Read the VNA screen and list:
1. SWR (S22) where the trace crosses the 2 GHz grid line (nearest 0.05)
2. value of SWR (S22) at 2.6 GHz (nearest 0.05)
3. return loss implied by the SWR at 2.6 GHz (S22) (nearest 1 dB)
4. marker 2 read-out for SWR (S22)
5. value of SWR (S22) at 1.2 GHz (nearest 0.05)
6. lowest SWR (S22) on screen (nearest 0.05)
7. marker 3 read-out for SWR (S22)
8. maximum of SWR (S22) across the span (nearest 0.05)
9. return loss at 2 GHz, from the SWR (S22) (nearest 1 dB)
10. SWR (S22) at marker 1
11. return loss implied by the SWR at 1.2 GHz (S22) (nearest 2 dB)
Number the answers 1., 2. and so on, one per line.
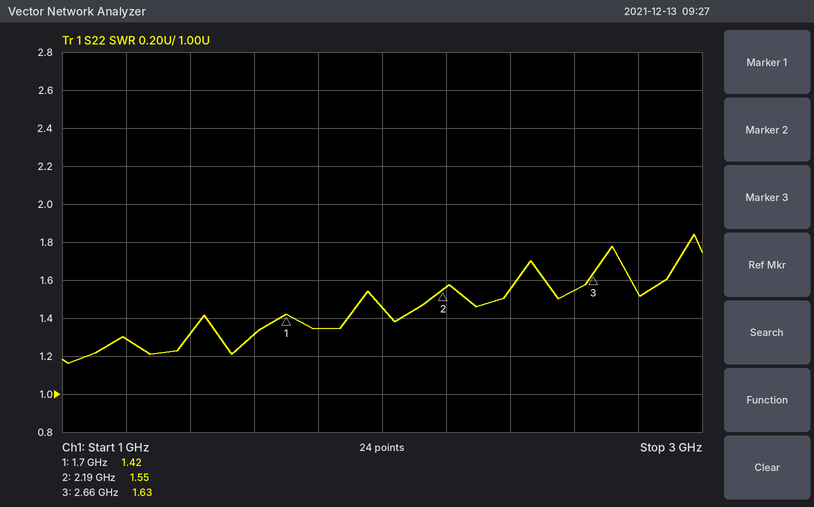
1. 1.45
2. 1.55
3. 13 dB
4. 1.55
5. 1.30
6. 1.15
7. 1.63
8. 1.85
9. 15 dB
10. 1.42
11. 18 dB
